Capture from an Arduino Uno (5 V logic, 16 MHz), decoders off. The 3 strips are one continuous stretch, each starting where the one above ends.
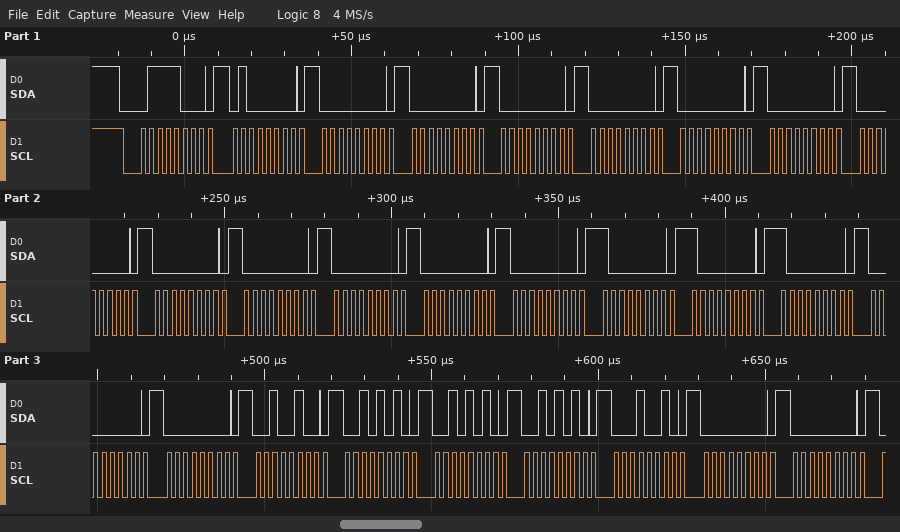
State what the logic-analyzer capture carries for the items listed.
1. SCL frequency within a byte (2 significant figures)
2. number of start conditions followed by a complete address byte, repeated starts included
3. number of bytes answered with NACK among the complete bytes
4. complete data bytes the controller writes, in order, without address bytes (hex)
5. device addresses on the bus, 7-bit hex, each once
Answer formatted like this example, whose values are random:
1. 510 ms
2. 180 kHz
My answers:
1. 400 kHz
2. 1
3. 0
4. 40 00 00 00 00 00 00 00 00 00 00 00 00 80 80 80 00 00 24 2A 2A 2A 12 00 00
5. 0x3C
